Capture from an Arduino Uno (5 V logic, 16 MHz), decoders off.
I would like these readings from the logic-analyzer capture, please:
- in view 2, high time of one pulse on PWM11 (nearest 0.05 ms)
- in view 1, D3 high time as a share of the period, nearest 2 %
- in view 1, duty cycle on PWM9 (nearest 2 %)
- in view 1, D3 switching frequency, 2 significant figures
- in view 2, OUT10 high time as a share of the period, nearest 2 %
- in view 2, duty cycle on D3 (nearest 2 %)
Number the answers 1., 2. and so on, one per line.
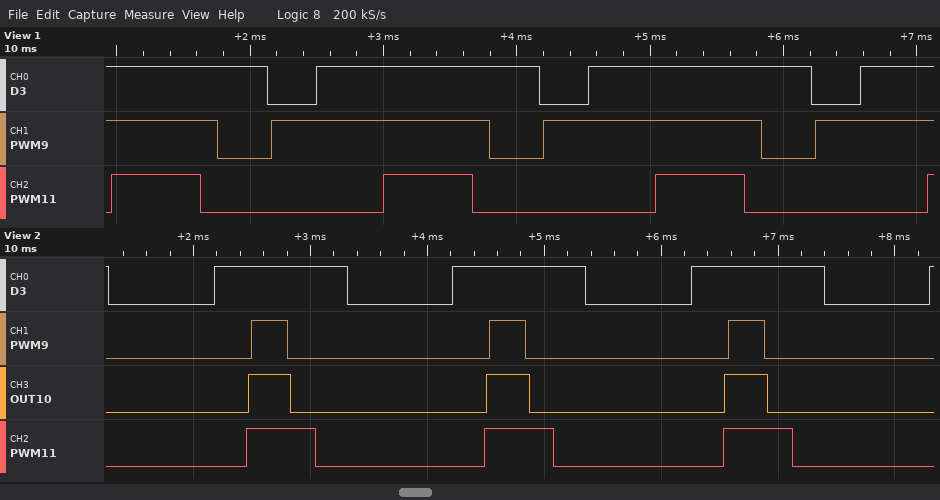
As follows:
1. 0.60 ms
2. 82 %
3. 80 %
4. 490 Hz
5. 18 %
6. 56 %
